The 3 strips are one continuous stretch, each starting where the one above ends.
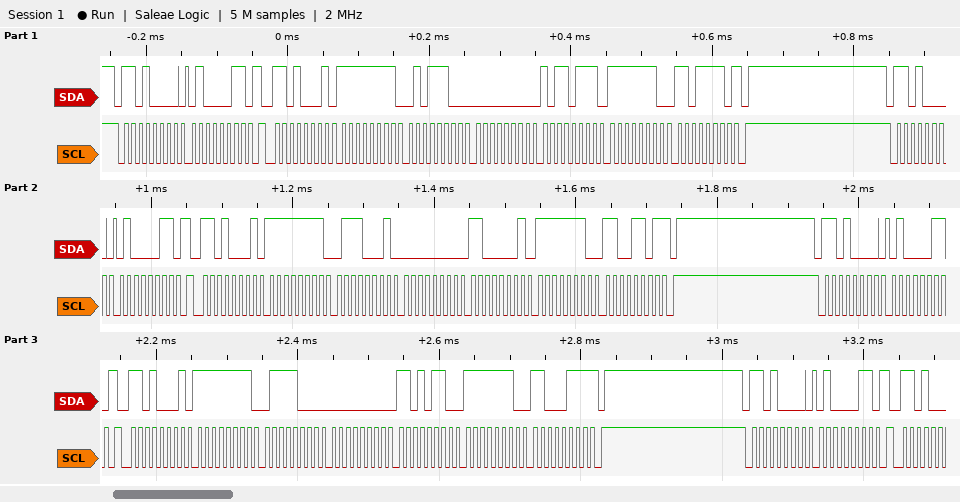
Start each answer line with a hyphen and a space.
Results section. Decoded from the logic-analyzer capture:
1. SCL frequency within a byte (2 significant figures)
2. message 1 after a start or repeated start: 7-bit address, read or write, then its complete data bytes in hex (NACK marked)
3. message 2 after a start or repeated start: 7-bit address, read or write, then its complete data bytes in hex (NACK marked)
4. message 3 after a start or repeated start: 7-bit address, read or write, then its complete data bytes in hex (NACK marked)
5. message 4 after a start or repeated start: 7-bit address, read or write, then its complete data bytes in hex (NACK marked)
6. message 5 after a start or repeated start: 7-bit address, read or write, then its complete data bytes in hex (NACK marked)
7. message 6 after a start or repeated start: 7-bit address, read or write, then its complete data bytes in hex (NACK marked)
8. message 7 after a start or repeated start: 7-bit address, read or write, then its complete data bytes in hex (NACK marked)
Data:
- 100 kHz
- 0x68 write: 43
- 0x68 read: FF 5C 00 B7 FE DE NACK
- 0x68 write: 43
- 0x68 read: FF 71 00 C1 FE CD NACK
- 0x68 write: 43
- 0x68 read: FF 78 00 D6 FE C7 NACK
- 0x68 write: 43
